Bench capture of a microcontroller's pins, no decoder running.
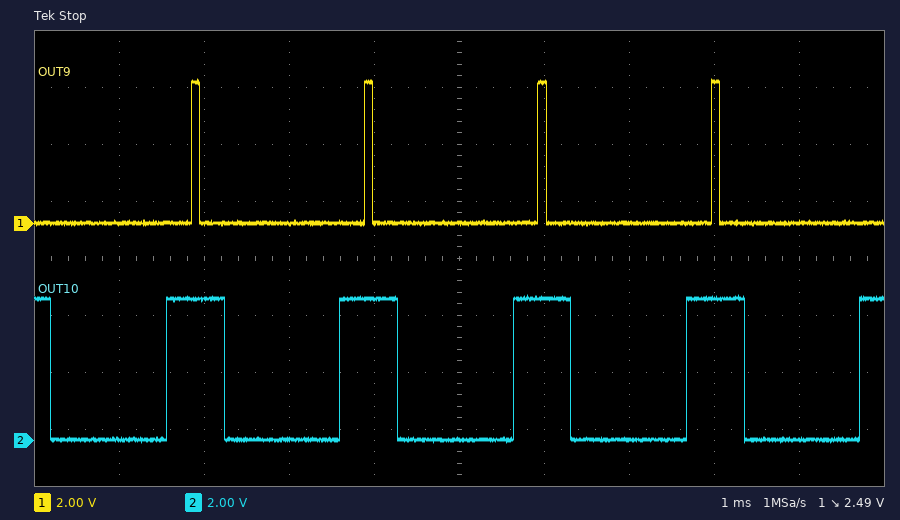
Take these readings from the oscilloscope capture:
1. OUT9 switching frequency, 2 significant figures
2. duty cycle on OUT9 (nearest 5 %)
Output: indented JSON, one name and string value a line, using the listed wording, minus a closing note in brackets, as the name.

{
  "OUT9 switching frequency, 2 significant figures": "490 Hz",
  "duty cycle on OUT9": "5 %"
}
